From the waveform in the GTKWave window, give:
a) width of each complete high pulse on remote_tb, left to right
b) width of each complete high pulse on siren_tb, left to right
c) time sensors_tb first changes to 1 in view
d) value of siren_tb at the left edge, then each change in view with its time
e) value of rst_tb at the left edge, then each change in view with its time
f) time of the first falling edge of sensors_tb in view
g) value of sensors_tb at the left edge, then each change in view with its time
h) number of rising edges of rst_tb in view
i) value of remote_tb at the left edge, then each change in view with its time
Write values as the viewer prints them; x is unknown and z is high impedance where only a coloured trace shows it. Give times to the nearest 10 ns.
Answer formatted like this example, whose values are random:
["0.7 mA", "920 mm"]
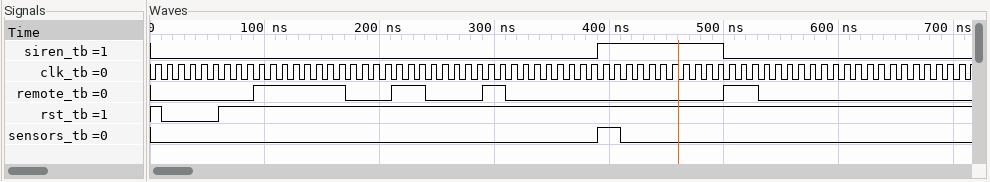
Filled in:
["80 ns, 30 ns, 20 ns, 30 ns", "110 ns", "390 ns", "0, 1 at 390 ns, 0 at 500 ns", "1, 0 at 10 ns, 1 at 60 ns", "410 ns", "0, 1 at 390 ns, 0 at 410 ns", "1", "0, 1 at 90 ns, 0 at 170 ns, 1 at 210 ns, 0 at 240 ns, 1 at 290 ns, 0 at 310 ns, 1 at 500 ns, 0 at 530 ns"]
